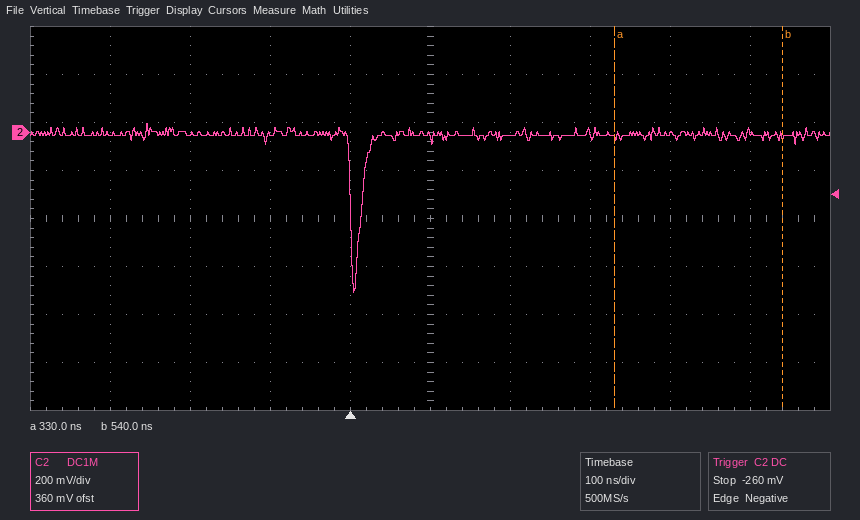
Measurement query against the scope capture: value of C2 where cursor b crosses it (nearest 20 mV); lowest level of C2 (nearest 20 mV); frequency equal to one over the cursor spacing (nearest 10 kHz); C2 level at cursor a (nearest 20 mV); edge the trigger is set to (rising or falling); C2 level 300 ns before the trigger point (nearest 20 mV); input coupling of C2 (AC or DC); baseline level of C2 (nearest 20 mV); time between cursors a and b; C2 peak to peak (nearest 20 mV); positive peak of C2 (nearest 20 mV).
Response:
-20 mV
-660 mV
4.76 MHz
-20 mV
falling
0 mV
DC
-20 mV
210 ns
700 mV
40 mV
